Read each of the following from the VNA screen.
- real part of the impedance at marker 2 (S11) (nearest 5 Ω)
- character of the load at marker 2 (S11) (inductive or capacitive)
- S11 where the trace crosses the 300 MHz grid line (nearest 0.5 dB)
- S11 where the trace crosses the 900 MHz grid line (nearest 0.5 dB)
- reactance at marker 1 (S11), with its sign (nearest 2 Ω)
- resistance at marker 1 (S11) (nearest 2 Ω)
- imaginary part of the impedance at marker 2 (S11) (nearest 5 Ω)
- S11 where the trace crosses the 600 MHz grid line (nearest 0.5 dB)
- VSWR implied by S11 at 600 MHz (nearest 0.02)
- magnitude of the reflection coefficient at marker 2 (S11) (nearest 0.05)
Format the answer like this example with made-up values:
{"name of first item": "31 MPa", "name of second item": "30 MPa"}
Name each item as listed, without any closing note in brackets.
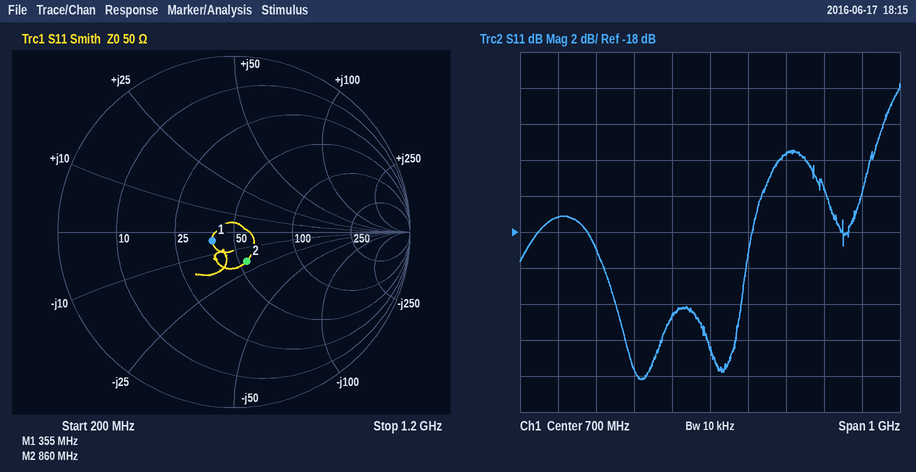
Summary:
{"real part of the impedance at marker 2 (S11)": "55 Ω", "character of the load at marker 2 (S11)": "capacitive", "S11 where the trace crosses the 300 MHz grid line": "-17.0 dB", "S11 where the trace crosses the 900 MHz grid line": "-13.5 dB", "reactance at marker 1 (S11), with its sign": "-4 Ω", "resistance at marker 1 (S11)": "38 Ω", "imaginary part of the impedance at marker 2 (S11)": "-20 Ω", "S11 where the trace crosses the 600 MHz grid line": "-22.5 dB", "VSWR implied by S11 at 600 MHz": "1.16", "magnitude of the reflection coefficient at marker 2 (S11)": "0.20"}
